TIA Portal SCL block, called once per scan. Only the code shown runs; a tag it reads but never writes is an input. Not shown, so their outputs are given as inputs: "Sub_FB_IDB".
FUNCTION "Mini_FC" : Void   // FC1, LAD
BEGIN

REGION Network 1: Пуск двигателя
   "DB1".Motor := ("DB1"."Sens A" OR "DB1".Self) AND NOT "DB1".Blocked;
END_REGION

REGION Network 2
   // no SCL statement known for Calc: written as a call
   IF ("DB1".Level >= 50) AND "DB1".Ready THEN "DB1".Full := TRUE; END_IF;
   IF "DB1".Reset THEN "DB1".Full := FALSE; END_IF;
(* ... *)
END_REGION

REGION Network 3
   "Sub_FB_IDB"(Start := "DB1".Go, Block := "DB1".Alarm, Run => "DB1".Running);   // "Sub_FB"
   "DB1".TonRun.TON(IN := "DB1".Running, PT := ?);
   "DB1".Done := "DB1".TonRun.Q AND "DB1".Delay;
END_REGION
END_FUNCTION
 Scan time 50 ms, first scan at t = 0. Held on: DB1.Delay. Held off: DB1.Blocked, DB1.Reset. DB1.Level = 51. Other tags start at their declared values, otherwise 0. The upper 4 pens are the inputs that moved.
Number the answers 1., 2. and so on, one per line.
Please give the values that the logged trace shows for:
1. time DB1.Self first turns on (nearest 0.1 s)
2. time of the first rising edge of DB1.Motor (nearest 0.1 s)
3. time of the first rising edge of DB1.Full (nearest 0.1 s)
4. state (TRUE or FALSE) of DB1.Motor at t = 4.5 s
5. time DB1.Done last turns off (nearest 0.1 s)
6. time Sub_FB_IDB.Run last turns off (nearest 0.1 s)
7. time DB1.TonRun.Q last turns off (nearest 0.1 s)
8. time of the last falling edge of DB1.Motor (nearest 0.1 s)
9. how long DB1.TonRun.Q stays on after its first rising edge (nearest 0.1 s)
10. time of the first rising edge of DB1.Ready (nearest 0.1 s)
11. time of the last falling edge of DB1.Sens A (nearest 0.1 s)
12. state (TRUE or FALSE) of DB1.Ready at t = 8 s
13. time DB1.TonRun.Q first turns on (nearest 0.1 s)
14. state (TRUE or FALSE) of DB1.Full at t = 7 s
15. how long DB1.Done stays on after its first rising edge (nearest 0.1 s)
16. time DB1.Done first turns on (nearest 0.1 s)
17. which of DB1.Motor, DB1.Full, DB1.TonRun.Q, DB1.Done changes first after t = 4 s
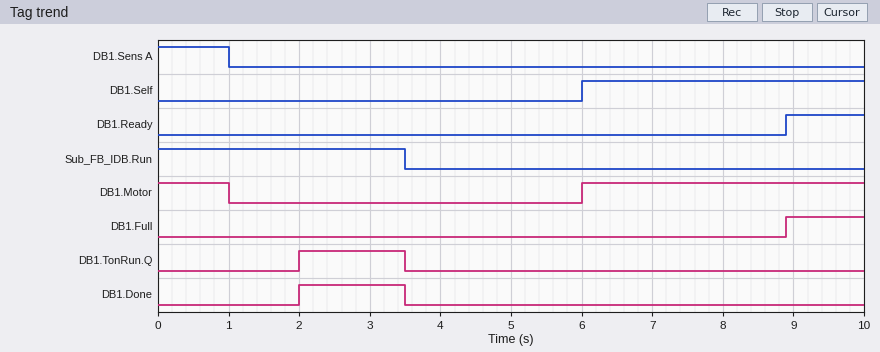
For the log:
1. 6.0 s
2. 6.0 s
3. 8.9 s
4. FALSE
5. 3.5 s
6. 3.5 s
7. 3.5 s
8. 1.0 s
9. 1.5 s
10. 8.9 s
11. 1.0 s
12. FALSE
13. 2.0 s
14. FALSE
15. 1.5 s
16. 2.0 s
17. DB1.Motor
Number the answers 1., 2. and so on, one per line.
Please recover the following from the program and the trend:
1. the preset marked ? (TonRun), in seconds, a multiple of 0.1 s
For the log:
1. 2.0 s
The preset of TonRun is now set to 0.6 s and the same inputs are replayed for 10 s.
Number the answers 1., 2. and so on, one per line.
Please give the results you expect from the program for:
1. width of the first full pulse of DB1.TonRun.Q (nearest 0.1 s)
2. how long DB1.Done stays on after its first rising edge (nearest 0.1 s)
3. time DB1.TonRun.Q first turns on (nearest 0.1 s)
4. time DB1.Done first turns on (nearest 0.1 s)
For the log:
1. 2.9 s
2. 2.9 s
3. 0.6 s
4. 0.6 s
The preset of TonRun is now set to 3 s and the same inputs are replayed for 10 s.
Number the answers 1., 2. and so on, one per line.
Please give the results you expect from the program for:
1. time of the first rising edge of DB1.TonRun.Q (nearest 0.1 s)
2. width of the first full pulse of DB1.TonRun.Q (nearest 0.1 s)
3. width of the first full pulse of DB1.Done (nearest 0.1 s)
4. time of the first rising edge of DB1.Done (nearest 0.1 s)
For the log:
1. 3.0 s
2. 0.5 s
3. 0.5 s
4. 3.0 s
